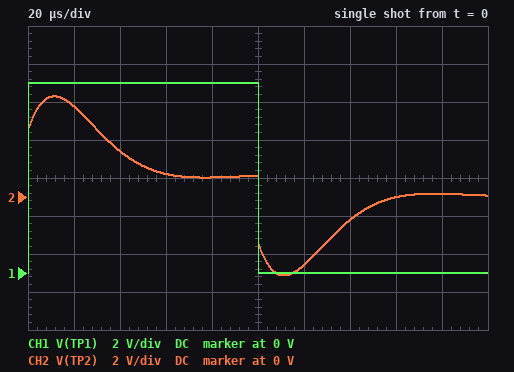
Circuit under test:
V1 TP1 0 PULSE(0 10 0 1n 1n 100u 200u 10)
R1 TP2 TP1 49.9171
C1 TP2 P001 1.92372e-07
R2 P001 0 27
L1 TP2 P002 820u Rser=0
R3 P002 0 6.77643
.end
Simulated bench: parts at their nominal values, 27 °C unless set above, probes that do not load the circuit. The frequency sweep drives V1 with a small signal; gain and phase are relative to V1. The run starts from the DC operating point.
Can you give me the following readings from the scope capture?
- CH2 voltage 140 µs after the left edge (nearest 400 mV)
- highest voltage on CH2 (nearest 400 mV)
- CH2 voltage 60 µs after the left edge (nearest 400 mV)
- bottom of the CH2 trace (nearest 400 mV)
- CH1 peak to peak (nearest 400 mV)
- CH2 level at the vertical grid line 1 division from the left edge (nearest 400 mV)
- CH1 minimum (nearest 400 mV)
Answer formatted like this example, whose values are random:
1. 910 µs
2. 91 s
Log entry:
1. -1.2 V
2. 5.2 V
3. 1.2 V
4. -4.0 V
5. 10.0 V
6. 4.8 V
7. 0 V
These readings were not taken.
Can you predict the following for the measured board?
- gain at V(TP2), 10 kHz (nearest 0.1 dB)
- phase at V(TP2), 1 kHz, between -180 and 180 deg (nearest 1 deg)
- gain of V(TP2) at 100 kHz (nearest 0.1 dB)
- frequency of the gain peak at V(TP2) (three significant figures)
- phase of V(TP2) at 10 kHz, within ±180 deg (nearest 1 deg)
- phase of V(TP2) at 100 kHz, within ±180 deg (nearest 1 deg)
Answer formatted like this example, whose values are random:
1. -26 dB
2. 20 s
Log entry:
1. -2.7 dB
2. 32 deg
3. -8.7 dB
4. 11.5 kHz
5. 17 deg
6. -9 deg
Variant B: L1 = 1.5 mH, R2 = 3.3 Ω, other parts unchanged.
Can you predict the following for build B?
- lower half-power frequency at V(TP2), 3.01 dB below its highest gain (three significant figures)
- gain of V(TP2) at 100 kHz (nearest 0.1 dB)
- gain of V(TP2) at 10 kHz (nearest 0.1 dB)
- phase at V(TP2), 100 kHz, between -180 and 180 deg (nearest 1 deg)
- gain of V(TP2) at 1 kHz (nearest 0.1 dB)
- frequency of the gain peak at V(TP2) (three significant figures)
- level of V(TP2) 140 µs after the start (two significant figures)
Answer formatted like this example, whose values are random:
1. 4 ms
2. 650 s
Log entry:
1. 4.39 kHz
2. -15.6 dB
3. -0.5 dB
4. -59 deg
5. -13.8 dB
6. 9.64 kHz
7. -3.3 V
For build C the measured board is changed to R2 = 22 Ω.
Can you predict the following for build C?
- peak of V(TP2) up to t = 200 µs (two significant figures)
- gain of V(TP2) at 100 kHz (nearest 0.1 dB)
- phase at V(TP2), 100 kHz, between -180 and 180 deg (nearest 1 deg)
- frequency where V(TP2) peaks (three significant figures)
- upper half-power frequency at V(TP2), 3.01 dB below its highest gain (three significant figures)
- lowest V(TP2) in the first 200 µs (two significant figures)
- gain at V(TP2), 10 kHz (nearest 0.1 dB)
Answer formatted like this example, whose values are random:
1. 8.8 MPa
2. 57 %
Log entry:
1. 5.4 V
2. -9.7 dB
3. -12 deg
4. 11.7 kHz
5. 25.1 kHz
6. -4.2 V
7. -2.5 dB
